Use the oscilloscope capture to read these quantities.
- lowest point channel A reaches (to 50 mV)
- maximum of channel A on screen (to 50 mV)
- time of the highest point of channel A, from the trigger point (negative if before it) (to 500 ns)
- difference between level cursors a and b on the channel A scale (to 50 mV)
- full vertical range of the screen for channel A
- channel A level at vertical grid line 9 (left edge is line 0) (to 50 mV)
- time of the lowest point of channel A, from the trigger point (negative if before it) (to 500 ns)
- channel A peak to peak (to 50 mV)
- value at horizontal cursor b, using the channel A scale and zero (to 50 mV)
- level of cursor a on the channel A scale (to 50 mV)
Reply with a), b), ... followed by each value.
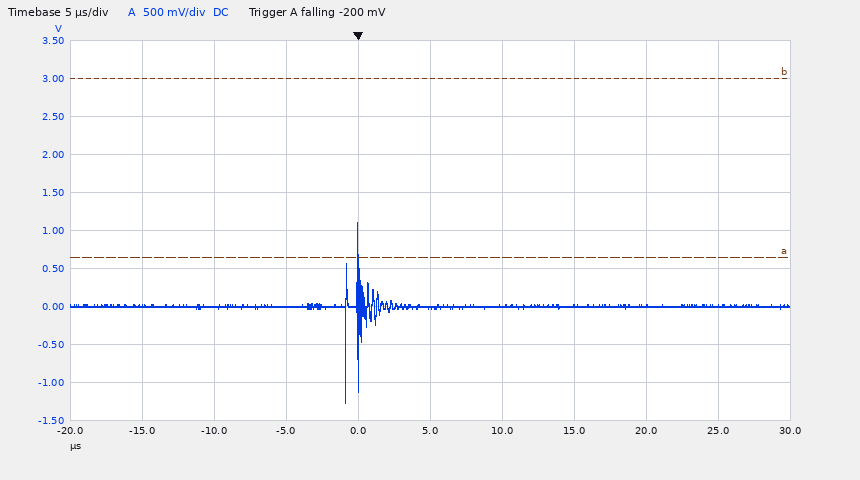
a) -1.25 V
b) 1.10 V
c) 0.0 µs
d) 2.35 V
e) 5 V
f) 0 mV
g) -1.0 µs
h) 2.35 V
i) 3.00 V
j) 650 mV
